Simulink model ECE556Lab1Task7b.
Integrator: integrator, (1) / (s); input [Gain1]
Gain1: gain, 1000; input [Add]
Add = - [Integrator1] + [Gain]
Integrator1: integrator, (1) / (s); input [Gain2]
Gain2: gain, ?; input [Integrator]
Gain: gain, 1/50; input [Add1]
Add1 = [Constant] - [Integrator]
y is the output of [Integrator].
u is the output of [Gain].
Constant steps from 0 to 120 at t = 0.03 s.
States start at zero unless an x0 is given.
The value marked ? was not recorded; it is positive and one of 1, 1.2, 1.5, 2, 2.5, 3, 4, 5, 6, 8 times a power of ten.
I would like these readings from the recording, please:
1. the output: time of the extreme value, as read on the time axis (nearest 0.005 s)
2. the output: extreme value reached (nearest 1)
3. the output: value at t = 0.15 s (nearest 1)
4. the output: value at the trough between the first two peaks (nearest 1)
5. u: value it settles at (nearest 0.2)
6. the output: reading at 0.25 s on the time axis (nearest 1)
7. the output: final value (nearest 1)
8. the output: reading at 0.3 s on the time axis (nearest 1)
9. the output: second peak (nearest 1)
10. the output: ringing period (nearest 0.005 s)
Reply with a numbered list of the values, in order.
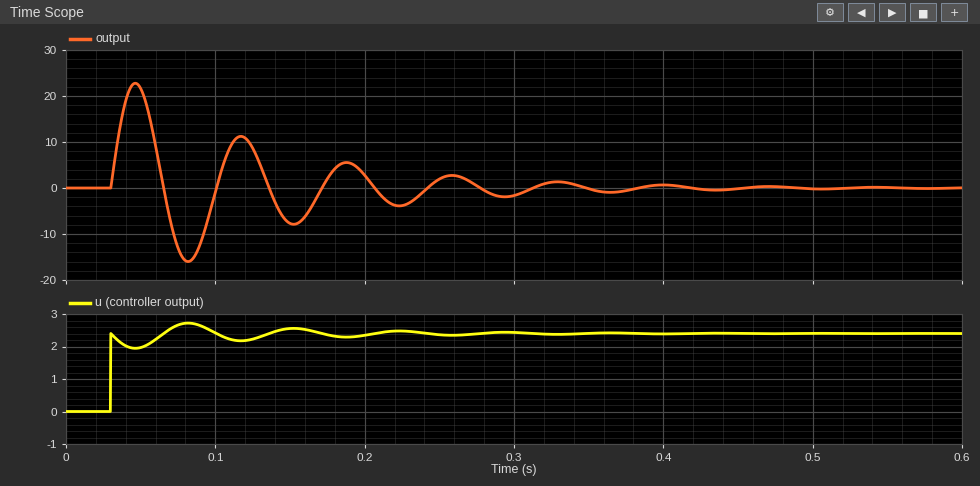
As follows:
1. 0.045 s
2. 23
3. -8
4. -16
5. 2.4
6. 2
7. 0
8. -2
9. 11
10. 0.070 s
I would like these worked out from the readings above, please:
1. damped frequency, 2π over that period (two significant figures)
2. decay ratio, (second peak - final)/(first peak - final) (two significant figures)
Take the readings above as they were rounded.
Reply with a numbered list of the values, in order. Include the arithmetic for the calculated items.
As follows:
1. 2π / 0.07 = 90 rad/s
2. (11 - 0) / (23 - 0) = 0.48
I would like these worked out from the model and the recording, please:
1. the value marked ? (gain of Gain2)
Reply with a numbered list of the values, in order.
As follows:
1. 8
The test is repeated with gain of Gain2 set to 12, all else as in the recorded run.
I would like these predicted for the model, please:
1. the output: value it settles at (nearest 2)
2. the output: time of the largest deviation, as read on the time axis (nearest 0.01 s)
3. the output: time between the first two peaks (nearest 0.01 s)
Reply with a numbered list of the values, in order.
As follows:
1. 0
2. 0.04 s
3. 0.06 s
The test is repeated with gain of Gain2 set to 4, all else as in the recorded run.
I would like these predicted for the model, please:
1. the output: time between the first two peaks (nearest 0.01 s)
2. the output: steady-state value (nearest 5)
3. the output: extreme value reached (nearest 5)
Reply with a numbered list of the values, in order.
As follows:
1. 0.10 s
2. 0
3. 30
